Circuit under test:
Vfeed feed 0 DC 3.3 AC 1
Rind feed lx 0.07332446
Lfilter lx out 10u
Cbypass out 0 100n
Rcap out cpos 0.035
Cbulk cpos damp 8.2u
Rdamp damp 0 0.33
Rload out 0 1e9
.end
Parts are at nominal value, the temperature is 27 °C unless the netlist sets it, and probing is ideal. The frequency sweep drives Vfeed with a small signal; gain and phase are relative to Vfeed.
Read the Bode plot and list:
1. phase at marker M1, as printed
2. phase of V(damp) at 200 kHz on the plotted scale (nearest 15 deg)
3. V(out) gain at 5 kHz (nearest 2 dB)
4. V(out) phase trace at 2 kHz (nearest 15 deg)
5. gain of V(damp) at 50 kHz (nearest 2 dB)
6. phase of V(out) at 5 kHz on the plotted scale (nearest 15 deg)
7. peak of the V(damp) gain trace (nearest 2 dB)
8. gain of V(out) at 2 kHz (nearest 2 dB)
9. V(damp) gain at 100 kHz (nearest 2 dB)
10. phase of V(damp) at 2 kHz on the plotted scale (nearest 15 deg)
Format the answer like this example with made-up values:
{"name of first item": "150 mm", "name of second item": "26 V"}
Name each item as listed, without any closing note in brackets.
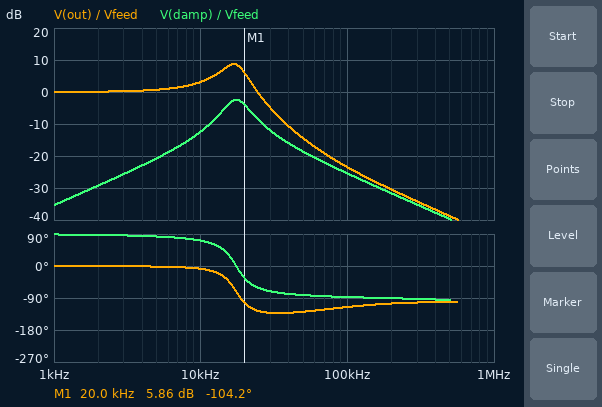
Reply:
{"phase at marker M1, as printed": "-104.2 deg", "phase of V(damp) at 200 kHz on the plotted scale": "-90 deg", "V(out) gain at 5 kHz": "0 dB", "V(out) phase trace at 2 kHz": "0 deg", "gain of V(damp) at 50 kHz": "-18 dB", "phase of V(out) at 5 kHz on the plotted scale": "0 deg", "peak of the V(damp) gain trace": "-2 dB", "gain of V(out) at 2 kHz": "0 dB", "V(damp) gain at 100 kHz": "-26 dB", "phase of V(damp) at 2 kHz on the plotted scale": "90 deg"}
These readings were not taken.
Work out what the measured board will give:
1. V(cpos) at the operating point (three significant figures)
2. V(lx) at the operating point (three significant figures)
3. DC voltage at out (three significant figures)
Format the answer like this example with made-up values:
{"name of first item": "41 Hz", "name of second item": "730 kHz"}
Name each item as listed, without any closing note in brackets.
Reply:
{"V(cpos) at the operating point": "3.30 V", "V(lx) at the operating point": "3.30 V", "DC voltage at out": "3.30 V"}
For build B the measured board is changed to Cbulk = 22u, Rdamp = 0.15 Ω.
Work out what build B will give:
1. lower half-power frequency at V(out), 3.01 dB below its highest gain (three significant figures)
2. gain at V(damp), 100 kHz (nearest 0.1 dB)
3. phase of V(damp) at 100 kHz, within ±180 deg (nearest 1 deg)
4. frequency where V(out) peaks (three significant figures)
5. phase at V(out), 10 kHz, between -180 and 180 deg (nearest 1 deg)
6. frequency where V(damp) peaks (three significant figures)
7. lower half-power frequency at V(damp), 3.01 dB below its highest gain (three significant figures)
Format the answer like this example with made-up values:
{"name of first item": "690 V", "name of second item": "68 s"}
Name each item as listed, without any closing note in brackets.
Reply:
{"lower half-power frequency at V(out), 3.01 dB below its highest gain": "8.03 kHz", "gain at V(damp), 100 kHz": "-32.4 dB", "phase of V(damp) at 100 kHz, within ±180 deg": "-88 deg", "frequency where V(out) peaks": "10.3 kHz", "phase at V(out), 10 kHz, between -180 and 180 deg": "-56 deg", "frequency where V(damp) peaks": "10.7 kHz", "lower half-power frequency at V(damp), 3.01 dB below its highest gain": "8.86 kHz"}
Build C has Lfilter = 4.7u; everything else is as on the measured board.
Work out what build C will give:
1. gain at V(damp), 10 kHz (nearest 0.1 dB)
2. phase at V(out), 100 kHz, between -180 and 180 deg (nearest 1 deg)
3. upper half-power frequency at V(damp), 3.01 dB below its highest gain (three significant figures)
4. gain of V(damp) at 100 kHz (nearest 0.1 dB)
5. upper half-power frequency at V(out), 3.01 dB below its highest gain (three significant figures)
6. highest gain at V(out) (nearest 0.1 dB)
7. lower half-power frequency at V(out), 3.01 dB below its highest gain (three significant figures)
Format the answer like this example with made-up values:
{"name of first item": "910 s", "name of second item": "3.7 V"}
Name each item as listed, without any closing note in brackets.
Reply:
{"gain at V(damp), 10 kHz": "-14.2 dB", "phase at V(out), 100 kHz, between -180 and 180 deg": "-110 deg", "upper half-power frequency at V(damp), 3.01 dB below its highest gain": "33.8 kHz", "gain of V(damp) at 100 kHz": "-18.6 dB", "upper half-power frequency at V(out), 3.01 dB below its highest gain": "30.7 kHz", "highest gain at V(out)": "6.0 dB", "lower half-power frequency at V(out), 3.01 dB below its highest gain": "15.0 kHz"}
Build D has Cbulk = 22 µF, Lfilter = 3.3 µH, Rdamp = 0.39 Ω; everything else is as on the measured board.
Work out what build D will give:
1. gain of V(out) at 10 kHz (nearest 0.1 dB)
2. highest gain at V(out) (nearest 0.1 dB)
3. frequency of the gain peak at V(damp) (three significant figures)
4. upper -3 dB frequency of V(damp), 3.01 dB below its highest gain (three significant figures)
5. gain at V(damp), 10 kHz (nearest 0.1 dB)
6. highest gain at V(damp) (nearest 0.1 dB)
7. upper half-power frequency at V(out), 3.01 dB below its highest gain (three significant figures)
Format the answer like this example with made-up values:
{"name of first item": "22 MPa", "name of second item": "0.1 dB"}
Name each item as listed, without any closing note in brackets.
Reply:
{"gain of V(out) at 10 kHz": "1.4 dB", "highest gain at V(out)": "1.8 dB", "frequency of the gain peak at V(damp)": "18.7 kHz", "upper -3 dB frequency of V(damp), 3.01 dB below its highest gain": "34.2 kHz", "gain at V(damp), 10 kHz": "-5.3 dB", "highest gain at V(damp)": "-2.1 dB", "upper half-power frequency at V(out), 3.01 dB below its highest gain": "27.2 kHz"}
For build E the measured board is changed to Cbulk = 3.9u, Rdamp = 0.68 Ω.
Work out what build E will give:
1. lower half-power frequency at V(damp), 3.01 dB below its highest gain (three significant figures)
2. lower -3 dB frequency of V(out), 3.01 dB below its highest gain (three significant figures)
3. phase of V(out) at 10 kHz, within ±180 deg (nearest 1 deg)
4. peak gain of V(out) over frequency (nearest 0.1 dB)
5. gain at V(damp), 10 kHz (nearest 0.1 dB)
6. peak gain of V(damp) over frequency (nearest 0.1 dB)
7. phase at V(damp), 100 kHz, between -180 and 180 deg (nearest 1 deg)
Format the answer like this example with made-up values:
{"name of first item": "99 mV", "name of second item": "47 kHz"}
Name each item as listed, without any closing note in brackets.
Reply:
{"lower half-power frequency at V(damp), 3.01 dB below its highest gain": "19.9 kHz", "lower -3 dB frequency of V(out), 3.01 dB below its highest gain": "17.1 kHz", "phase of V(out) at 10 kHz, within ±180 deg": "-3 deg", "peak gain of V(out) over frequency": "7.4 dB", "gain at V(damp), 10 kHz": "-14.3 dB", "peak gain of V(damp) over frequency": "-1.1 dB", "phase at V(damp), 100 kHz, between -180 and 180 deg": "-85 deg"}
